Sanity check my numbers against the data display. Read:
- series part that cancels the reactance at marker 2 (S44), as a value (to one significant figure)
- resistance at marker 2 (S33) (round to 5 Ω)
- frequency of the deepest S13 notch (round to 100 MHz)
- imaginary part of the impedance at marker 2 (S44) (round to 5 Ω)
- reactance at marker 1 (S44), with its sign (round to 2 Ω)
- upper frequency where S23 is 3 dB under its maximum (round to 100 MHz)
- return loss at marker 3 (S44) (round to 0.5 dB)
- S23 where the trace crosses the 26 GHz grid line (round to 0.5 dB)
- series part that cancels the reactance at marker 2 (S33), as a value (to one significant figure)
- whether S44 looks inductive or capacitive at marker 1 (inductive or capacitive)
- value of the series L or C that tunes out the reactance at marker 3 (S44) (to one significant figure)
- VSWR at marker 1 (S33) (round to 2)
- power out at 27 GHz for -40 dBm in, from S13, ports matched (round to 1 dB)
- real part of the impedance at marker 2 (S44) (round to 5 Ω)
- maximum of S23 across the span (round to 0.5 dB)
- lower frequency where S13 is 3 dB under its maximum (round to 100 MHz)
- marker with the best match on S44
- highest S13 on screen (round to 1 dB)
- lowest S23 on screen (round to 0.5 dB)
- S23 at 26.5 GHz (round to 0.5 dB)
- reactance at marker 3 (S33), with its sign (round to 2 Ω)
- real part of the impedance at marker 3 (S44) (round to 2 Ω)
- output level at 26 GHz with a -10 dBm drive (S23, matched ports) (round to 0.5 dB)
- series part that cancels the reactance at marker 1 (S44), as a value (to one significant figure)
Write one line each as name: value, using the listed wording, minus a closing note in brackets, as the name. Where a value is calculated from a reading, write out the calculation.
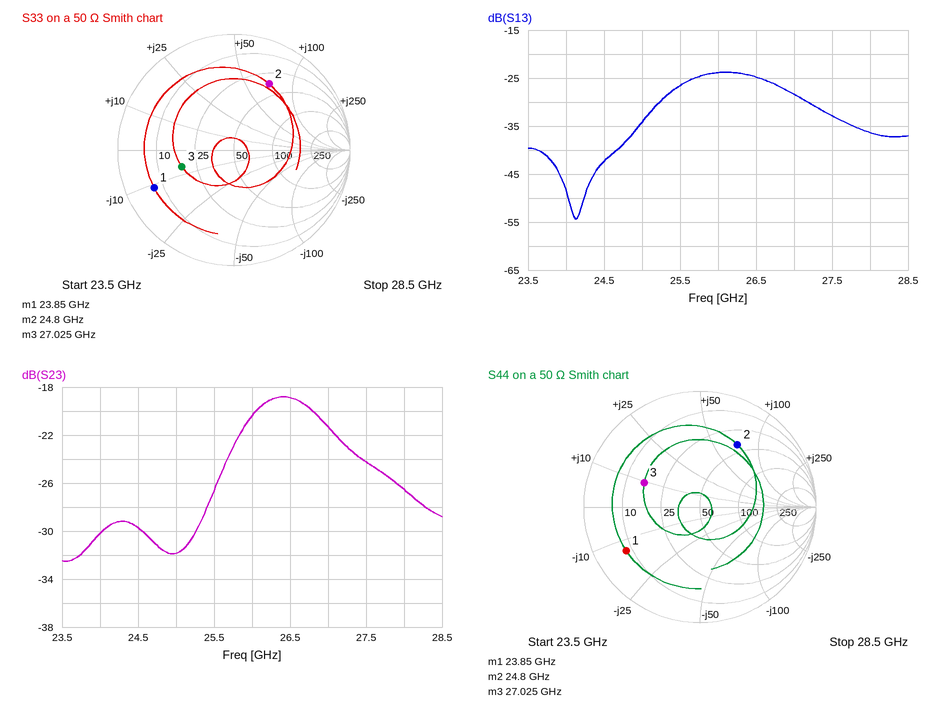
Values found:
series part that cancels the reactance at marker 2 (S44), as a value: C = 1/(2π × 24.8 GHz × 70 Ω) ≈ 91.7 fF, so 90 fF to one significant figure
resistance at marker 2 (S33): 35 Ω
frequency of the deepest S13 notch: 24.1 GHz
imaginary part of the impedance at marker 2 (S44): +70 Ω
reactance at marker 1 (S44), with its sign: -14 Ω
upper frequency where S23 is 3 dB under its maximum: 27.1 GHz
return loss at marker 3 (S44): 5.5 dB
S23 where the trace crosses the 26 GHz grid line: -20.5 dB
series part that cancels the reactance at marker 2 (S33), as a value: C = 1/(2π × 24.8 GHz × 70 Ω) ≈ 91.7 fF, so 90 fF to one significant figure
whether S44 looks inductive or capacitive at marker 1: capacitive
value of the series L or C that tunes out the reactance at marker 3 (S44): C = 1/(2π × 27.025 GHz × 10 Ω) ≈ 589 fF, so 600 fF to one significant figure
VSWR at marker 1 (S33): 8
power out at 27 GHz for -40 dBm in, from S13, ports matched: -40 dBm + (-28 dB) = -68 dBm
real part of the impedance at marker 2 (S44): 40 Ω
maximum of S23 across the span: -19.0 dB
lower frequency where S13 is 3 dB under its maximum: 25.5 GHz
marker with the best match on S44: marker 3
highest S13 on screen: -24 dB
lowest S23 on screen: -32.5 dB
S23 at 26.5 GHz: -19.0 dB
reactance at marker 3 (S33), with its sign: -6 Ω
real part of the impedance at marker 3 (S44): 16 Ω
output level at 26 GHz with a -10 dBm drive (S23, matched ports): -10 dBm + (-20.5 dB) = -30.5 dBm
series part that cancels the reactance at marker 1 (S44), as a value: L = 14 Ω/(2π × 23.85 GHz) ≈ 93.4 pH, so 90 pH to one significant figure
